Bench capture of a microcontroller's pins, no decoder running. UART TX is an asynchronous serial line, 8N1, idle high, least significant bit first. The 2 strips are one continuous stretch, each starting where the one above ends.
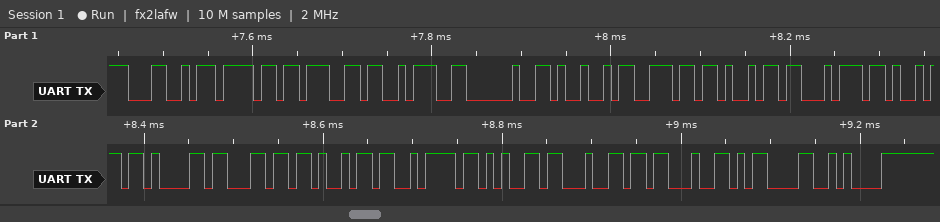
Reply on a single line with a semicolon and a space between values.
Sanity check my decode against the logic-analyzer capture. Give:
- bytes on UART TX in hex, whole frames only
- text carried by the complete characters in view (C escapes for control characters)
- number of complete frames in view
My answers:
4C 6F 67 3A 20 49 6E 69 74 69 61 6C 69 7A 65 64 23 0D 0A; "Log: Initialized#\r\n"; 19
